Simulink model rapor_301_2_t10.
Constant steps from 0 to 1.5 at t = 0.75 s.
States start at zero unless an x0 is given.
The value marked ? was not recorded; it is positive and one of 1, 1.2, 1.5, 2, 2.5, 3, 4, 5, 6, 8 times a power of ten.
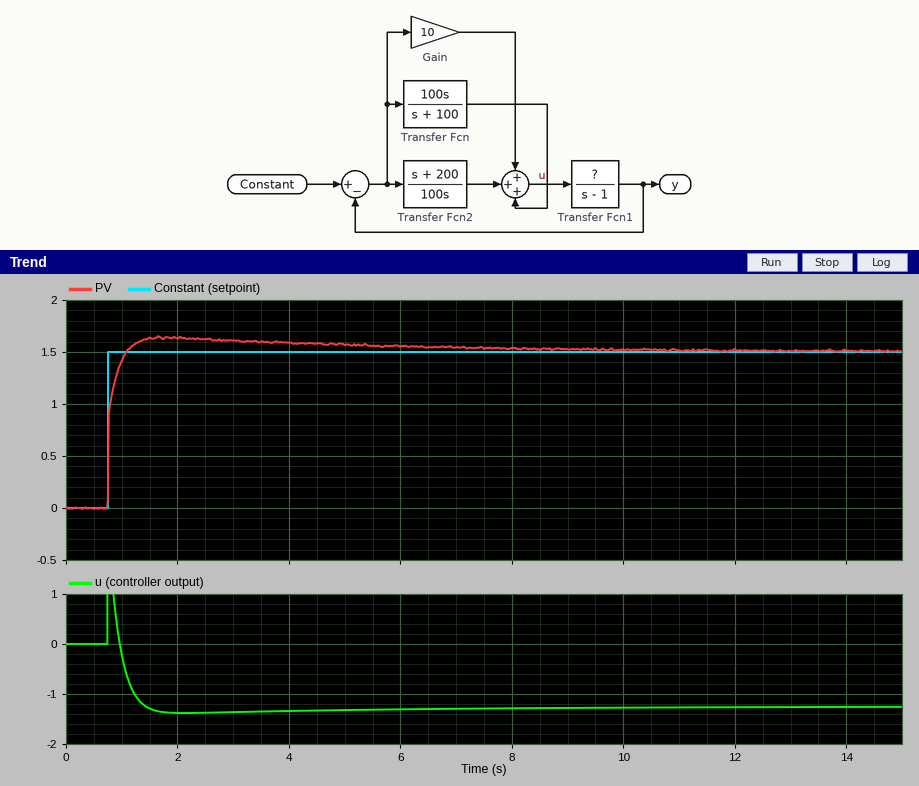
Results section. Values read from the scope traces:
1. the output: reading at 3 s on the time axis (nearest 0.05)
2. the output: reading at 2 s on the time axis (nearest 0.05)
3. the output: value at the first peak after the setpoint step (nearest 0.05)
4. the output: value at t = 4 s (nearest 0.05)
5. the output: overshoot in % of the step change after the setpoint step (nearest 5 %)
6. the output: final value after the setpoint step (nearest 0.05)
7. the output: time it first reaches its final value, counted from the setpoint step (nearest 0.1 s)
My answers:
1.60
1.65
1.65
1.60
10 %
1.50
0.3 s
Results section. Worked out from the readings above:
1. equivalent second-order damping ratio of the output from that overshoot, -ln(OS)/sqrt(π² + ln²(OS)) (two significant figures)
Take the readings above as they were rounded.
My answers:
0.59
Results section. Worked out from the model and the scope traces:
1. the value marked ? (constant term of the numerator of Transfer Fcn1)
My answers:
1.2
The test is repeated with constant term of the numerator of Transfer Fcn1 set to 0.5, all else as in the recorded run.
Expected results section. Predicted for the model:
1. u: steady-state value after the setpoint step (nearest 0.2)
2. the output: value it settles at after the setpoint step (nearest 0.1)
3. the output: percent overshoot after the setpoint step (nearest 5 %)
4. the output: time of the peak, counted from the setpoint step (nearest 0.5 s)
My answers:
-3.0
1.5
25 %
1.5 s
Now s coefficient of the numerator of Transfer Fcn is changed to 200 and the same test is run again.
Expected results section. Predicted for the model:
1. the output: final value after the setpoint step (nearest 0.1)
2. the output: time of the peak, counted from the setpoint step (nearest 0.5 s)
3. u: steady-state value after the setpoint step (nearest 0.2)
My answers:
1.5
1.5 s
-1.2
